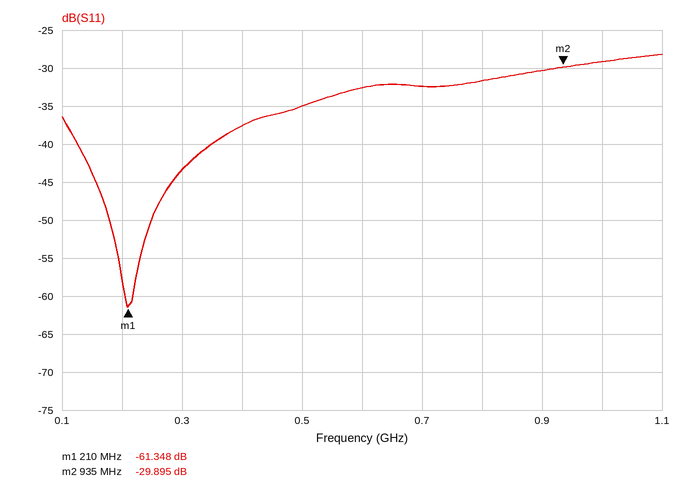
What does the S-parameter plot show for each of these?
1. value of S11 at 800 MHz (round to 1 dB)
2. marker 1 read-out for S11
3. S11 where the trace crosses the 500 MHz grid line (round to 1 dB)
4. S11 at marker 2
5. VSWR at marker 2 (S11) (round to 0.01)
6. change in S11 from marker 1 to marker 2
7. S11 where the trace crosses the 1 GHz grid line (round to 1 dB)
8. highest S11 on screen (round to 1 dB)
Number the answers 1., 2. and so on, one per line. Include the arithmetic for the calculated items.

1. -32 dB
2. -61.348 dB
3. -35 dB
4. -29.895 dB
5. (1 + 0.0320)/(1 − 0.0320) ≈ 1.07
6. -29.895 − (-61.348) = 31.453 dB
7. -29 dB
8. -28 dB
